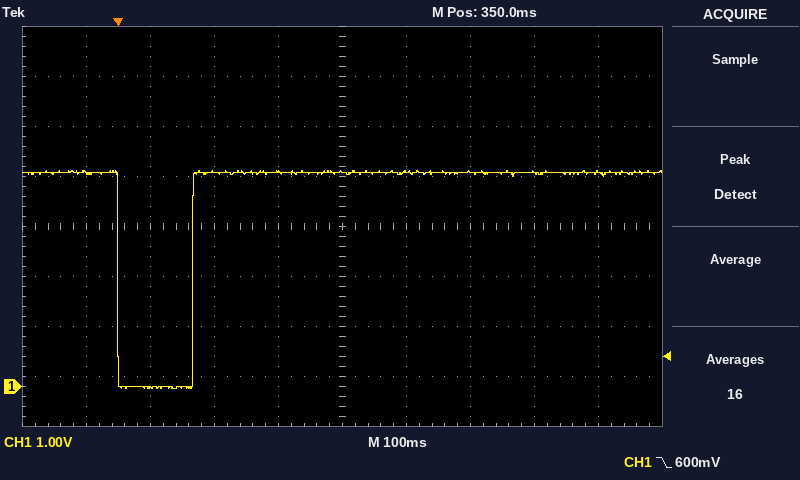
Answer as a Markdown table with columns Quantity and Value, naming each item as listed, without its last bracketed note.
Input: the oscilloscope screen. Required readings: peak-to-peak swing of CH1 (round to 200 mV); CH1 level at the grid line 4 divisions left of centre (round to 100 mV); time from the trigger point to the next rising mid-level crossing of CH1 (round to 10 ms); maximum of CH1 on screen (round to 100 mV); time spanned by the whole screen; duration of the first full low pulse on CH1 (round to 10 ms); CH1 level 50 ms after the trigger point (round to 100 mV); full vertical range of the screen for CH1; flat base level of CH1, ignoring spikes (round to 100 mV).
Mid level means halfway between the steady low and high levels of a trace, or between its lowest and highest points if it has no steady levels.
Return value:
| Quantity | Value |
|---|---|
| peak-to-peak swing of CH1 | 4.4 V |
| CH1 level at the grid line 4 divisions left of centre | 4.3 V |
| time from the trigger point to the next rising mid-level crossing of CH1 | 120 ms |
| maximum of CH1 on screen | 4.3 V |
| time spanned by the whole screen | 1 s |
| duration of the first full low pulse on CH1 | 120 ms |
| CH1 level 50 ms after the trigger point | 0.0 V |
| full vertical range of the screen for CH1 | 8 V |
| flat base level of CH1, ignoring spikes | 0.0 V |
